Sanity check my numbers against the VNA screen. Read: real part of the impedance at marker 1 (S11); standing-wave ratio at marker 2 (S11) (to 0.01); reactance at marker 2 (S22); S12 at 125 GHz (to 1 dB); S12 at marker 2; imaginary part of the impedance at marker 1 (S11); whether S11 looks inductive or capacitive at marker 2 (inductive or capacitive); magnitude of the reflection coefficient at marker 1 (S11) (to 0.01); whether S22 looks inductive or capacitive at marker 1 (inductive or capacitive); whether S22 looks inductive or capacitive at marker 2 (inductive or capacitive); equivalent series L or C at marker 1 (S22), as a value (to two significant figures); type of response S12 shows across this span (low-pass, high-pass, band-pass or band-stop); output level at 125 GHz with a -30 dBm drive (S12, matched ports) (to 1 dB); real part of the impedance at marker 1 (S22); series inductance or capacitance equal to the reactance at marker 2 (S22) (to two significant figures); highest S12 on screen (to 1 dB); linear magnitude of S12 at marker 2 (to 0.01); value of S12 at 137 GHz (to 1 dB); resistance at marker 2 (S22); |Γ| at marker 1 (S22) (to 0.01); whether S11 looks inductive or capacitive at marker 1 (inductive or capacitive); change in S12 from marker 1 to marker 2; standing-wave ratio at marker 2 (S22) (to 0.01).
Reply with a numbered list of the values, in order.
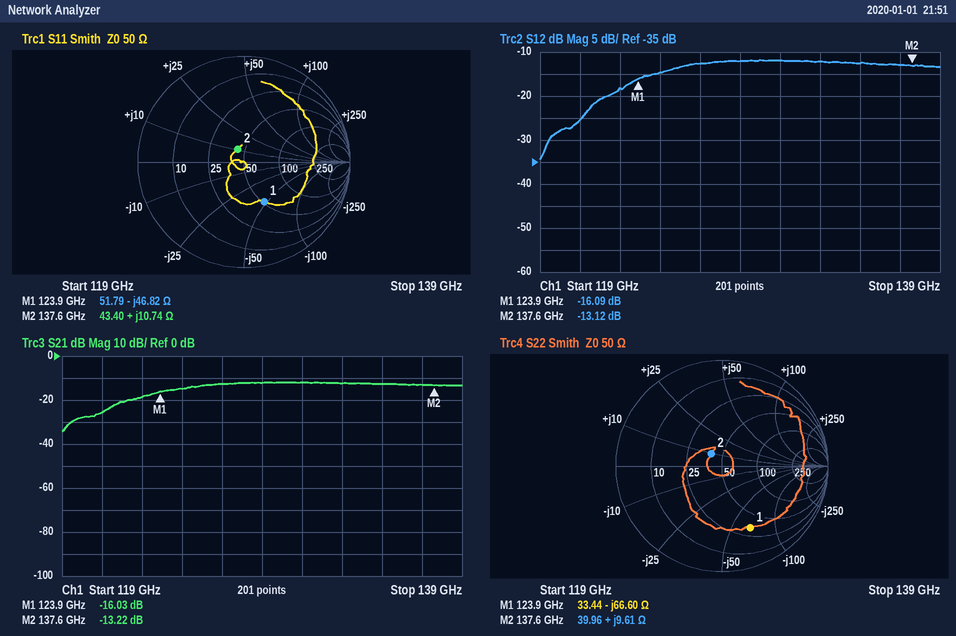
1. 51.79 Ω
2. 1.31
3. +9.61 Ω
4. -15 dB
5. -13.12 dB
6. -46.82 Ω
7. inductive
8. 0.42
9. capacitive
10. inductive
11. 19 fF
12. high-pass
13. -45 dBm
14. 33.44 Ω
15. 11 pH
16. -12 dB
17. 0.22
18. -13 dB
19. 39.96 Ω
20. 0.64
21. capacitive
22. 2.97 dB
23. 1.36
